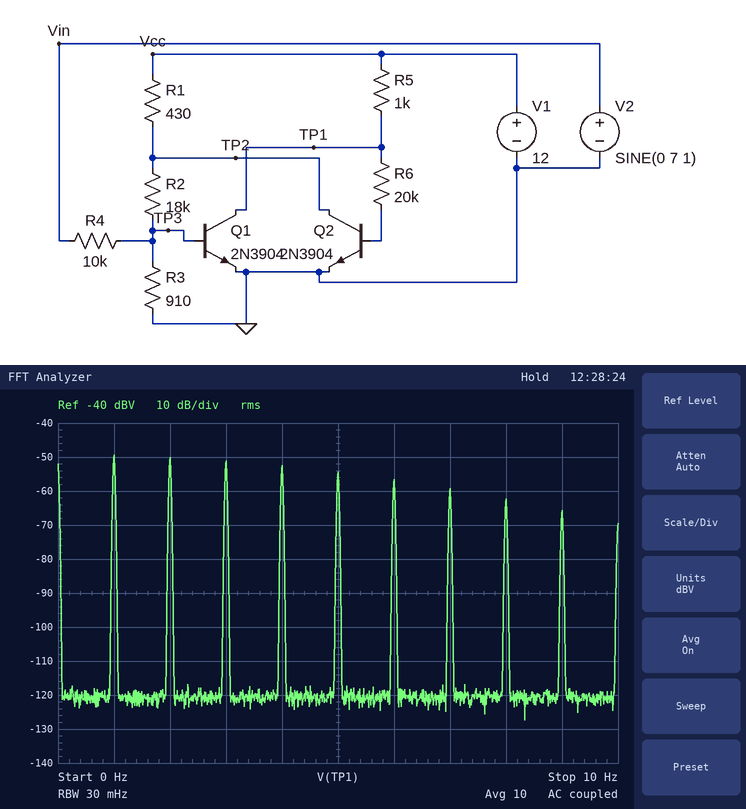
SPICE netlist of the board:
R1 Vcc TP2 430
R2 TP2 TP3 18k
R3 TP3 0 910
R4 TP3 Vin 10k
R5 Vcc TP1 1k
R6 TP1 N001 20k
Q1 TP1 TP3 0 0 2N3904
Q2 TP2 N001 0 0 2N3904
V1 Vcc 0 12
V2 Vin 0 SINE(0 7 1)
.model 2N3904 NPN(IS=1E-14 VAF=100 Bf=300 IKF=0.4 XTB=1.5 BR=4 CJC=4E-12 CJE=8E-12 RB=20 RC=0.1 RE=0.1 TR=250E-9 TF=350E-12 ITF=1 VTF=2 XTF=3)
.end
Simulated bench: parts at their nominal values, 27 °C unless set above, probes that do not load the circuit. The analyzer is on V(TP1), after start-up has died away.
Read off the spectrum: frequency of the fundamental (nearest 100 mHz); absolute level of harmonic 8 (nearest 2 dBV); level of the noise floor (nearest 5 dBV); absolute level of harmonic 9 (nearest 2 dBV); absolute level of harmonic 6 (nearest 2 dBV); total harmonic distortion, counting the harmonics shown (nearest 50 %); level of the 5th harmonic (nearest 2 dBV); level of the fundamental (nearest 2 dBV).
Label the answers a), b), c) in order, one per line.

a) 1.0 Hz
b) -62 dBV
c) -120 dBV
d) -66 dBV
e) -56 dBV
f) 150 %
g) -54 dBV
h) -50 dBV
